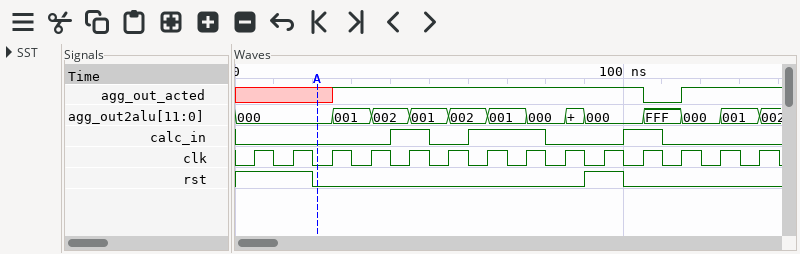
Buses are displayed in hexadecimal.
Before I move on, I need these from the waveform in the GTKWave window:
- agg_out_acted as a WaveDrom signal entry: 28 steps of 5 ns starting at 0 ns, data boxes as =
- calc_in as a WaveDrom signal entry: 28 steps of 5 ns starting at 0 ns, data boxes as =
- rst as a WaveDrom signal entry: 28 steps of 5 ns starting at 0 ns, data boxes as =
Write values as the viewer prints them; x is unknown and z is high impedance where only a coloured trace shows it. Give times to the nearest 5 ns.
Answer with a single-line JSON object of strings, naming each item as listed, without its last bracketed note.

{"agg_out_acted as a WaveDrom signal entry: 28 steps of 5 ns starting at 0 ns, data boxes as =": "{name: 'agg_out_acted', wave: 'x....1...............0.1....'}", "calc_in as a WaveDrom signal entry: 28 steps of 5 ns starting at 0 ns, data boxes as =": "{name: 'calc_in', wave: '0.......1.0.1...0...1.0.....'}", "rst as a WaveDrom signal entry: 28 steps of 5 ns starting at 0 ns, data boxes as =": "{name: 'rst', wave: '1...0.............1.0.......'}"}
